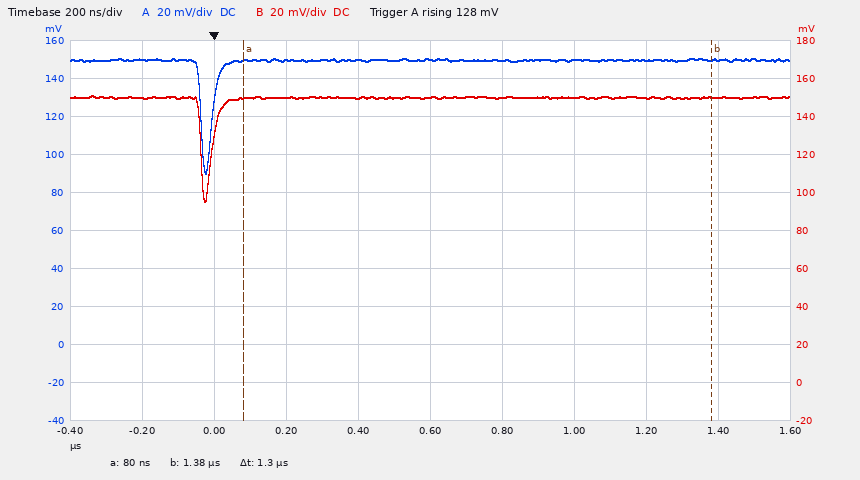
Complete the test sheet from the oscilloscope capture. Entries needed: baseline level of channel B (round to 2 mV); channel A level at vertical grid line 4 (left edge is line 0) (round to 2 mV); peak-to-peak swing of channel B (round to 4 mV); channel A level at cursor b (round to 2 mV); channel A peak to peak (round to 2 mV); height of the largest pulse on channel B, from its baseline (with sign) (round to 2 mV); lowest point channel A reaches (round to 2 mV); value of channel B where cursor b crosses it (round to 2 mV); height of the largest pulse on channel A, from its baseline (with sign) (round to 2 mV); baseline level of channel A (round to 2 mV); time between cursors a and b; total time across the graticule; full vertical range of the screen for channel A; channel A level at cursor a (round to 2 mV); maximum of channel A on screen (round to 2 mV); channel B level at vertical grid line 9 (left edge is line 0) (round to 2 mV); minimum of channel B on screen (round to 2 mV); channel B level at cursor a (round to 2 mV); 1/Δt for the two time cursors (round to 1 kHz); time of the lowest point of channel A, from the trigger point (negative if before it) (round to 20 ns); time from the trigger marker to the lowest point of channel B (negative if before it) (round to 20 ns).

150 mV
150 mV
56 mV
150 mV
60 mV
-54 mV
90 mV
150 mV
-60 mV
150 mV
1.3 µs
2 µs
200 mV
150 mV
150 mV
150 mV
96 mV
150 mV
769 kHz
-20 ns
-20 ns
